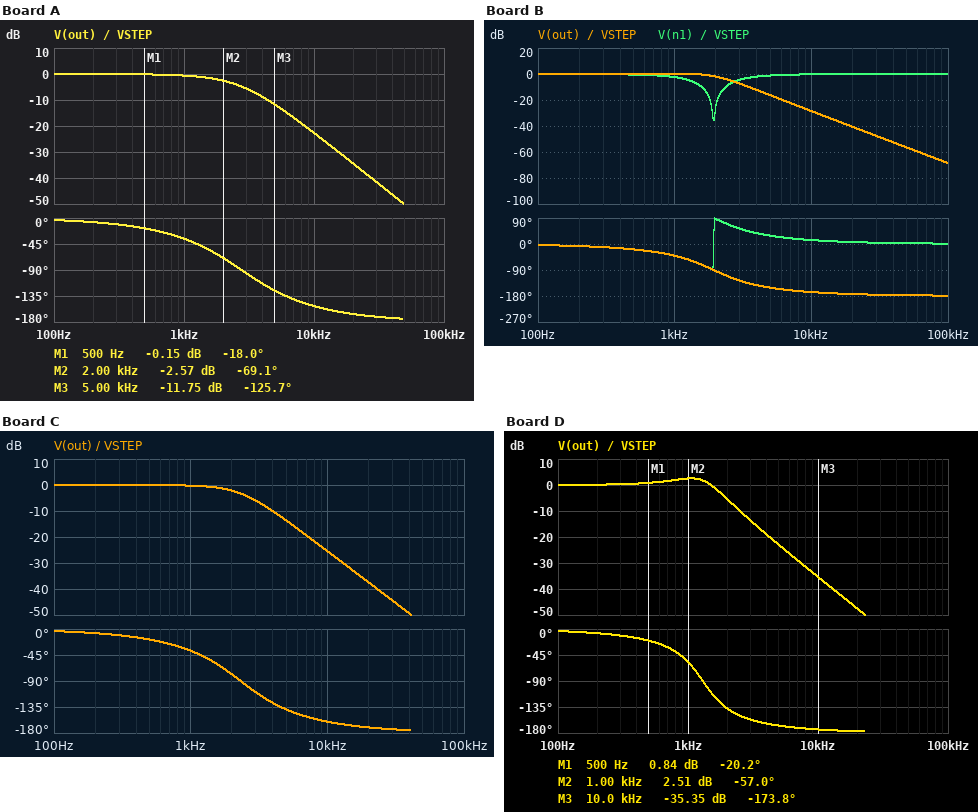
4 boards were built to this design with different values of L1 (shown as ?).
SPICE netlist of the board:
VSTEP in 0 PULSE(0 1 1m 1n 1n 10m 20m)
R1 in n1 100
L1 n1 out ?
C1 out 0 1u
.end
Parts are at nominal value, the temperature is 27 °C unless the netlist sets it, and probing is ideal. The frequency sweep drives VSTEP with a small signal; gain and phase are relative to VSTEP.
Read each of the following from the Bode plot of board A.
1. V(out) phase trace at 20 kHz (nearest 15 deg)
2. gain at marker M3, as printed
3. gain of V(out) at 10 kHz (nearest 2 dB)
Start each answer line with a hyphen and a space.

- -165 deg
- -11.75 dB
- -22 dB
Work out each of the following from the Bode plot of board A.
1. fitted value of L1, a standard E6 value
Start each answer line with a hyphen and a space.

- 3.3 mH
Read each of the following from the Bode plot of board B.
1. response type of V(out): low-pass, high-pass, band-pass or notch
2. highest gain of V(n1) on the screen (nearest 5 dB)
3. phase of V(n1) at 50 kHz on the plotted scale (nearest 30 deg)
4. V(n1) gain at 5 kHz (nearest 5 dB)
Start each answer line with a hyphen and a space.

- low-pass
- 0 dB
- 0 deg
- 0 dB
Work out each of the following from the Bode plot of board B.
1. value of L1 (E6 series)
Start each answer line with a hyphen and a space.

- 6.8 mH
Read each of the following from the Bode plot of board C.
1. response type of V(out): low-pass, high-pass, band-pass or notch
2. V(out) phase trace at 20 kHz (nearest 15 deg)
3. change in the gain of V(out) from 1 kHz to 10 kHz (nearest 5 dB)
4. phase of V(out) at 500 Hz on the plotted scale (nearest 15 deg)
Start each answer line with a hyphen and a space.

- low-pass
- -165 deg
- -25 dB
- -15 deg
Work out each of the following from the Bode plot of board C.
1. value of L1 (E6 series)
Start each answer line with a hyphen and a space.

- 4.7 mH
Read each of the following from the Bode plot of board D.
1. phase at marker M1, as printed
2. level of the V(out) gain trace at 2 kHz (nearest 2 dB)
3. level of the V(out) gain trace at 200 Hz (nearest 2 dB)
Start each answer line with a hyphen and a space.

- -20.2 deg
- -6 dB
- 0 dB
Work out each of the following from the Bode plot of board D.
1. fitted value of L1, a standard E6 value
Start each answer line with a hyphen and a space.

- 15 mH
